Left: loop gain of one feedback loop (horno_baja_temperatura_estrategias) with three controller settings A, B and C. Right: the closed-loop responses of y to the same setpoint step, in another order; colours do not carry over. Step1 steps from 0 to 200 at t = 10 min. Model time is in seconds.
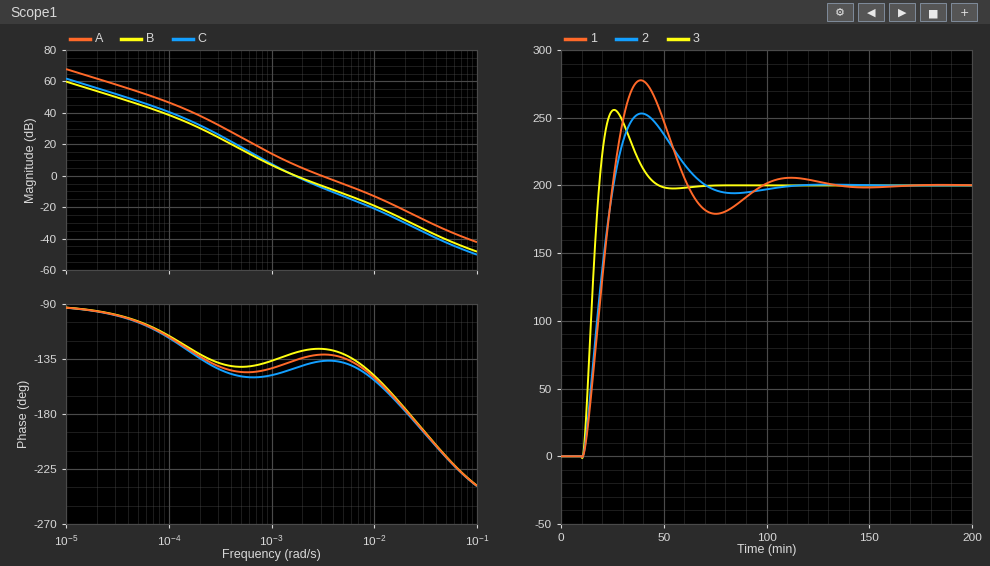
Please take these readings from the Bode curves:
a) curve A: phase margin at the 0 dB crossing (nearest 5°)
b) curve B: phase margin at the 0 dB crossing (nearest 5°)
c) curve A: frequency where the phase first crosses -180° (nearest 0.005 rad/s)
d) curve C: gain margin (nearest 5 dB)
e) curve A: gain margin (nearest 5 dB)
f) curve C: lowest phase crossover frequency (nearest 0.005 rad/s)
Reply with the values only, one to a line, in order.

50°
50°
0.020 rad/s
30 dB
25 dB
0.020 rad/s
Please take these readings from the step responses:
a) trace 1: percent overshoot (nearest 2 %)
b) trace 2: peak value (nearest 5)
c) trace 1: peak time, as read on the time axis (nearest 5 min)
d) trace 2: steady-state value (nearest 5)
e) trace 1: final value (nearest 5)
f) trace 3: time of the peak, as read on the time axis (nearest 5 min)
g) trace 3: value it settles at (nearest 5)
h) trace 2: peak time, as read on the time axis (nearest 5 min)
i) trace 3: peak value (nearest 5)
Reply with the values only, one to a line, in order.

38 %
255
40 min
200
200
25 min
200
40 min
255
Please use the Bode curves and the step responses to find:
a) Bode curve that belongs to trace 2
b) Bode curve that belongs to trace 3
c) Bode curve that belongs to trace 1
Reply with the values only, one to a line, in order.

B
A
C
